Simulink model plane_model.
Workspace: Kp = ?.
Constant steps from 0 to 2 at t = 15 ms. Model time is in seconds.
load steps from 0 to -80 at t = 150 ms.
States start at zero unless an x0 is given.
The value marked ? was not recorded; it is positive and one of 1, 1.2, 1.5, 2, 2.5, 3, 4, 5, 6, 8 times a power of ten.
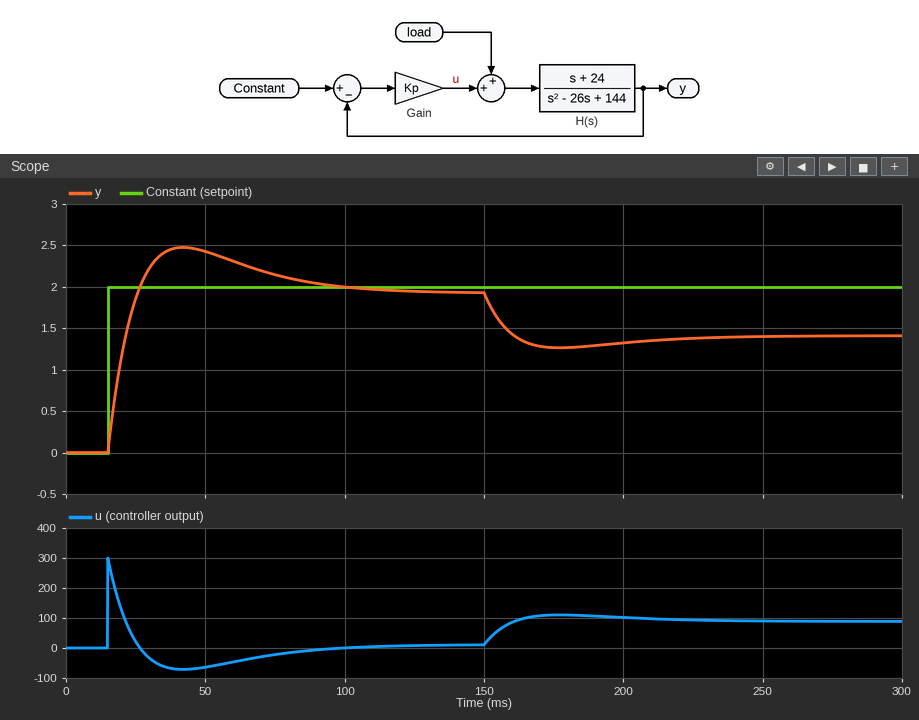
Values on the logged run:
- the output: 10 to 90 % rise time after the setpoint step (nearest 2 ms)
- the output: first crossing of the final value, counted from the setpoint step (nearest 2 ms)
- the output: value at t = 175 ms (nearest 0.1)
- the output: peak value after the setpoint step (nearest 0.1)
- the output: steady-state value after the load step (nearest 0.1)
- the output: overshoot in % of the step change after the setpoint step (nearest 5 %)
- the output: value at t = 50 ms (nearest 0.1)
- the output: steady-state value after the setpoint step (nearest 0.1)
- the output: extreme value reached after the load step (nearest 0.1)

8 ms
10 ms
1.3
2.5
1.4
30 %
2.4
1.9
1.3
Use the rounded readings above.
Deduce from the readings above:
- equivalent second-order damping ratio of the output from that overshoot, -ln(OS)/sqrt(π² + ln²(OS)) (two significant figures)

0.36
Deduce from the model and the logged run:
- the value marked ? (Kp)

150
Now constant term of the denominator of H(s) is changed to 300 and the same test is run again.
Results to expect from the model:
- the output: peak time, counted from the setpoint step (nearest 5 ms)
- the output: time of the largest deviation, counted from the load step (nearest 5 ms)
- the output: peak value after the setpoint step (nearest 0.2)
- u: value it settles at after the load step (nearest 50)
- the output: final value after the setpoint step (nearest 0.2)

25 ms
25 ms
2.4
100
1.8
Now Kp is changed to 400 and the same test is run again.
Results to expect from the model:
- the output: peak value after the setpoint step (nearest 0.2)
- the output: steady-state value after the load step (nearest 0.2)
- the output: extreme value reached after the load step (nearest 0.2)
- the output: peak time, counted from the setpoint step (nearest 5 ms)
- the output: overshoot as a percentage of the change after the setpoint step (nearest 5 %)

2.2
1.8
1.8
15 ms
10 %
